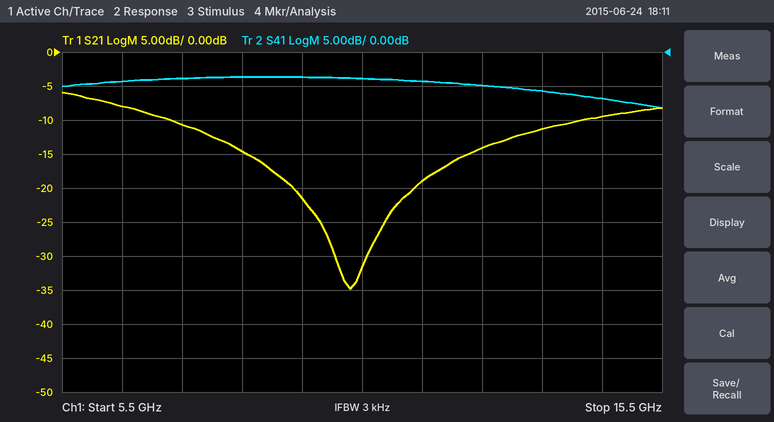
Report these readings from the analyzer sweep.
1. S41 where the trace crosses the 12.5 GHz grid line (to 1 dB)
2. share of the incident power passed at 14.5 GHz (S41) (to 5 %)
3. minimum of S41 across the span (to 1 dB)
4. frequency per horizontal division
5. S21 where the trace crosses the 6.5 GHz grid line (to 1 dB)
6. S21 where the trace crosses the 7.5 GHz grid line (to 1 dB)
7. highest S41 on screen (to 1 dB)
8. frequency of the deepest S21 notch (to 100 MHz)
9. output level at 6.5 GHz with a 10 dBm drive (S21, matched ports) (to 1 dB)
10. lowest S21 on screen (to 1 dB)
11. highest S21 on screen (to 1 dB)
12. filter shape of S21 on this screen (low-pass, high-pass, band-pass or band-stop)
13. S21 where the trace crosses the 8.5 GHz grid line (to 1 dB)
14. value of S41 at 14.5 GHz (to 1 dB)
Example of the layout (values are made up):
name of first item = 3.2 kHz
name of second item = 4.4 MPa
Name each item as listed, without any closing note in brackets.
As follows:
S41 where the trace crosses the 12.5 GHz grid line = -5 dB
share of the incident power passed at 14.5 GHz (S41) = 20 %
minimum of S41 across the span = -8 dB
frequency per horizontal division = 1 GHz
S21 where the trace crosses the 6.5 GHz grid line = -8 dB
S21 where the trace crosses the 7.5 GHz grid line = -11 dB
highest S41 on screen = -4 dB
frequency of the deepest S21 notch = 10.3 GHz
output level at 6.5 GHz with a 10 dBm drive (S21, matched ports) = 2 dBm
lowest S21 on screen = -35 dB
highest S21 on screen = -6 dB
filter shape of S21 on this screen = band-stop
S21 where the trace crosses the 8.5 GHz grid line = -15 dB
value of S41 at 14.5 GHz = -7 dB
